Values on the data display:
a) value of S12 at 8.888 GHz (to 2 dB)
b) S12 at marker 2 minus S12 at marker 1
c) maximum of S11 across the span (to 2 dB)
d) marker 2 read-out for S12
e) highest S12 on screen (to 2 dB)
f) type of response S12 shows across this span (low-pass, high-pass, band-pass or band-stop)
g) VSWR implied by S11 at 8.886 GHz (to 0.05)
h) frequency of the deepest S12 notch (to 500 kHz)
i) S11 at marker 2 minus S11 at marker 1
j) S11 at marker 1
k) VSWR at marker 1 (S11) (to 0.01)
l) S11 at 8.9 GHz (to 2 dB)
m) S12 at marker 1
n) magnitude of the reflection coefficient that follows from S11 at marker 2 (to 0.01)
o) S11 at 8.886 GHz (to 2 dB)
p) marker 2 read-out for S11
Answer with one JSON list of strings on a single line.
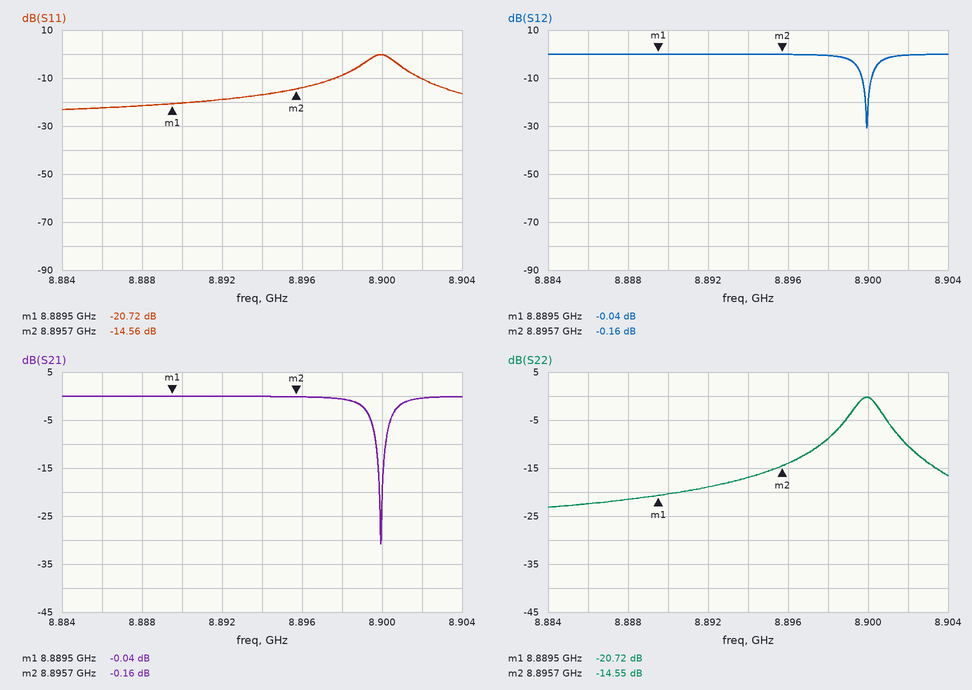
["0 dB", "-0.12 dB", "0 dB", "-0.16 dB", "0 dB", "band-stop", "1.15", "8.9000 GHz", "6.16 dB", "-20.72 dB", "1.20", "0 dB", "-0.04 dB", "0.19", "-22 dB", "-14.56 dB"]
